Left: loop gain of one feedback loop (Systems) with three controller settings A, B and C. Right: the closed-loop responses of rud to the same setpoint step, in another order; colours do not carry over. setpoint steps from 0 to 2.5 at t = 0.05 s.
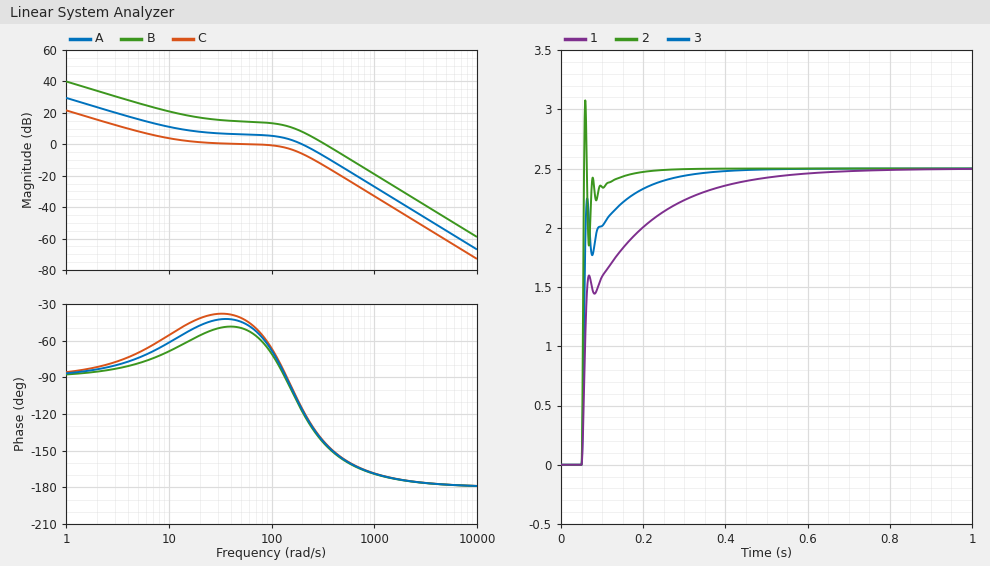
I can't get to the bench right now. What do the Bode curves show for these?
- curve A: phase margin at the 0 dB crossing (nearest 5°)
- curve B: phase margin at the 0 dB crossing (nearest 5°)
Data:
65°
35°
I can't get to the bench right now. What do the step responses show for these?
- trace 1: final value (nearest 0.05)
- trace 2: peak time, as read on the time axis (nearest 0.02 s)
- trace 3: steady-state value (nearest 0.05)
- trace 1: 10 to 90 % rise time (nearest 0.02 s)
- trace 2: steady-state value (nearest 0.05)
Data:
2.50
0.06 s
2.50
0.26 s
2.50
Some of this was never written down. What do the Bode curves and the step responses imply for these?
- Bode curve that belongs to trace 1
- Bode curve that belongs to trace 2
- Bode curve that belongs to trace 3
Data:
C
B
A
